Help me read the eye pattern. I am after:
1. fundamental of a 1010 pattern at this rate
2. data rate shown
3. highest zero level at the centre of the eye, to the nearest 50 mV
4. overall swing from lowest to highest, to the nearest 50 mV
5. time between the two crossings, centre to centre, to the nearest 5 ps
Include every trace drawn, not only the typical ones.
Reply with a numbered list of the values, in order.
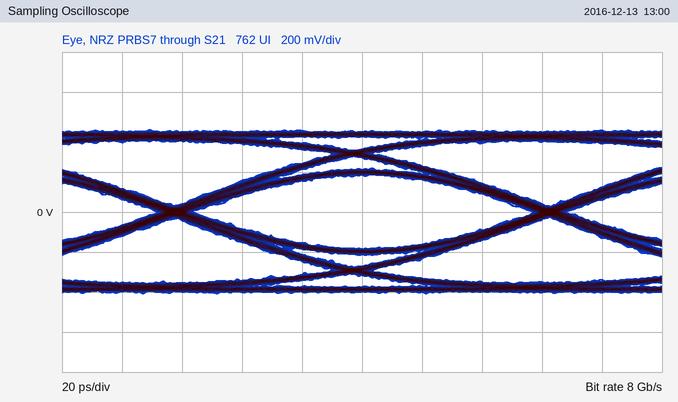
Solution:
1. 4 GHz
2. 8 Gb/s
3. -200 mV
4. 800 mV
5. 125 ps
